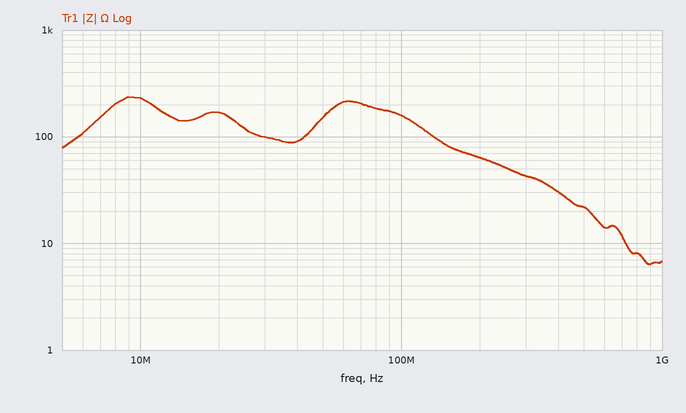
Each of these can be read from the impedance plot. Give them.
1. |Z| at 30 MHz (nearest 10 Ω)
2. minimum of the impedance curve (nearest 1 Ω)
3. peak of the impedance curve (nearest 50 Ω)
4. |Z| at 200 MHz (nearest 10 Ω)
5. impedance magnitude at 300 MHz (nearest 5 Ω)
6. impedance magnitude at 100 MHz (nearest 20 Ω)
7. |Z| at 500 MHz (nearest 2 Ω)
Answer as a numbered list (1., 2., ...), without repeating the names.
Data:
1. 100 Ω
2. 6 Ω
3. 250 Ω
4. 60 Ω
5. 45 Ω
6. 160 Ω
7. 22 Ω
